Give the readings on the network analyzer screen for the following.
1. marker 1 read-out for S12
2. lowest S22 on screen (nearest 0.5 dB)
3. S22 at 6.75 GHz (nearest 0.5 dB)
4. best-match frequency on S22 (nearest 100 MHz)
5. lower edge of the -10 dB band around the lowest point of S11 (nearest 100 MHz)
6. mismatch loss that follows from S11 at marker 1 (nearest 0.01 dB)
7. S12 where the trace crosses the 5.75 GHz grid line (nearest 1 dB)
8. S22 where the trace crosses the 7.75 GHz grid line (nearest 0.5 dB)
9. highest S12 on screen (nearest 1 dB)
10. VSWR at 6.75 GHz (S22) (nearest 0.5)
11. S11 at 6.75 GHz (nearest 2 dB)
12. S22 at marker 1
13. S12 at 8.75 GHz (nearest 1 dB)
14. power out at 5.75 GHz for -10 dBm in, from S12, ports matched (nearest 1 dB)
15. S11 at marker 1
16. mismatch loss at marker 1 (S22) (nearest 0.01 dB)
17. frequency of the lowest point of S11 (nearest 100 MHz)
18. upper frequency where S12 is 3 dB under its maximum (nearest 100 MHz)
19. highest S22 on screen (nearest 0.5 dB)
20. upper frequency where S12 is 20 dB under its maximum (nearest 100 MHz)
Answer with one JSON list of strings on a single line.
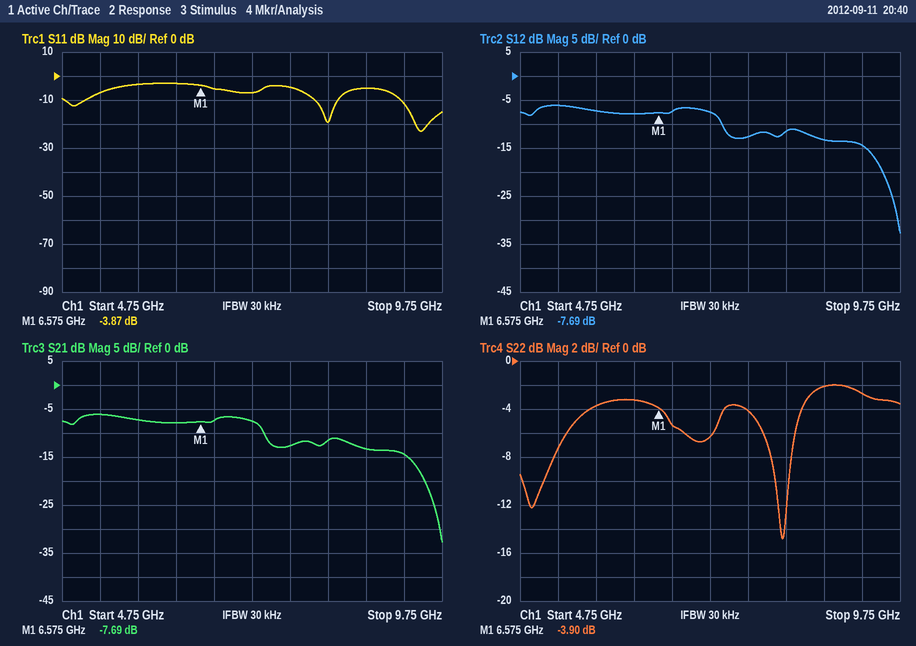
["-7.69 dB", "-15.0 dB", "-5.5 dB", "8.2 GHz", "9.2 GHz", "2.29 dB", "-7 dB", "-4.0 dB", "-6 dB", "3.5", "-6 dB", "-3.90 dB", "-13 dB", "-17 dBm", "-3.87 dB", "2.27 dB", "9.5 GHz", "7.4 GHz", "-2.0 dB", "9.7 GHz"]
